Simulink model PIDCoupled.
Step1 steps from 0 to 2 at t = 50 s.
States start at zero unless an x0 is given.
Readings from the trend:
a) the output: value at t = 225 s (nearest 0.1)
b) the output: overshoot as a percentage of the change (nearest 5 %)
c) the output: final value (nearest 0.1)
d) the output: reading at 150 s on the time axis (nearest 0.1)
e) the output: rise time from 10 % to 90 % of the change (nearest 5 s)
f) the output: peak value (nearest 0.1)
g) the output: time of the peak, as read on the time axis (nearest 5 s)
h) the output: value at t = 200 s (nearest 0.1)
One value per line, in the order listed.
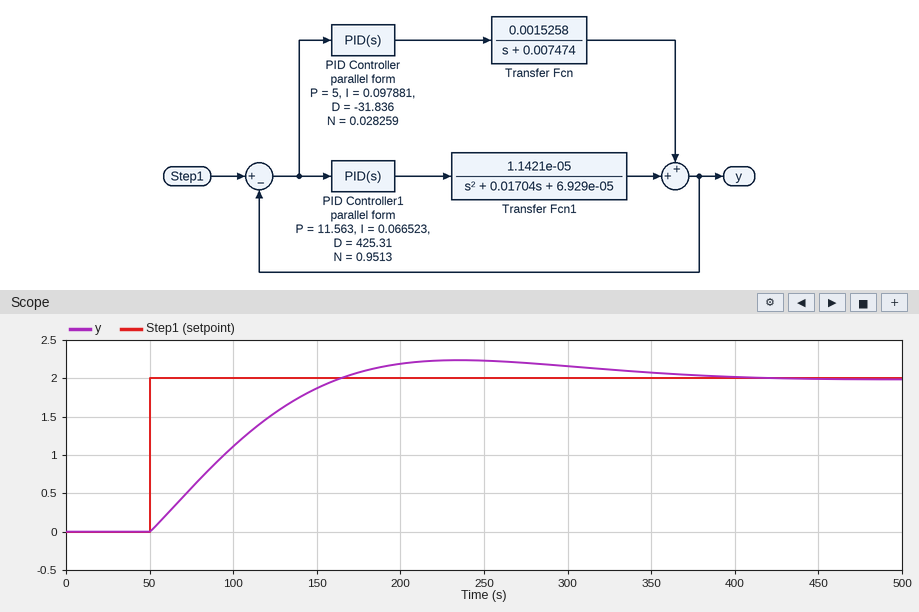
2.2
10 %
2.0
1.9
85 s
2.2
235 s
2.2
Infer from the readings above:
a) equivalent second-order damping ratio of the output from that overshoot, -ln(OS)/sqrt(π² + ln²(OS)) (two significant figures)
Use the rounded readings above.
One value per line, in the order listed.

0.59
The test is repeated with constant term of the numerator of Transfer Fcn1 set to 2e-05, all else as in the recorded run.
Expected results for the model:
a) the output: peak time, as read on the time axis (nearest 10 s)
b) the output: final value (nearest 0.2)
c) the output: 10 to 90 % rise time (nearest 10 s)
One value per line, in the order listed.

210 s
2.0
70 s
